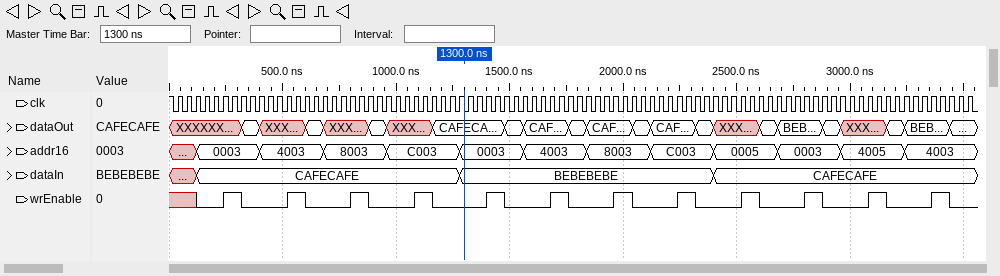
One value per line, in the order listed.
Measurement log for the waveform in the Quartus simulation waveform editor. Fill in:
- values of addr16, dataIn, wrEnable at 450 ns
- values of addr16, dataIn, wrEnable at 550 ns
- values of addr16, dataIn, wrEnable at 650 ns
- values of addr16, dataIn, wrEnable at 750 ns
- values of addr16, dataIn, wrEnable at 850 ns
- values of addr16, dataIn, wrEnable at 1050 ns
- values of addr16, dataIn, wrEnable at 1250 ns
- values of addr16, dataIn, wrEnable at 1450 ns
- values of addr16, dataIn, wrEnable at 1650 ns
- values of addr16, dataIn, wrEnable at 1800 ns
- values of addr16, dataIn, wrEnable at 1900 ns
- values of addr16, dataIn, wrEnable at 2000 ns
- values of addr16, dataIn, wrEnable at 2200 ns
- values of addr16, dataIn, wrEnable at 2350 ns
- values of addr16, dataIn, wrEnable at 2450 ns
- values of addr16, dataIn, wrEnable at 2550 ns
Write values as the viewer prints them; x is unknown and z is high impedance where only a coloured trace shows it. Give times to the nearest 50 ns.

addr16=4003, dataIn=CAFECAFE, wrEnable=0
addr16=4003, dataIn=CAFECAFE, wrEnable=1
addr16=4003, dataIn=CAFECAFE, wrEnable=0
addr16=8003, dataIn=CAFECAFE, wrEnable=0
addr16=8003, dataIn=CAFECAFE, wrEnable=1
addr16=C003, dataIn=CAFECAFE, wrEnable=0
addr16=C003, dataIn=CAFECAFE, wrEnable=0
addr16=0003, dataIn=BEBEBEBE, wrEnable=1
addr16=4003, dataIn=BEBEBEBE, wrEnable=0
addr16=4003, dataIn=BEBEBEBE, wrEnable=0
addr16=8003, dataIn=BEBEBEBE, wrEnable=0
addr16=8003, dataIn=BEBEBEBE, wrEnable=1
addr16=C003, dataIn=BEBEBEBE, wrEnable=0
addr16=C003, dataIn=BEBEBEBE, wrEnable=0
addr16=0005, dataIn=CAFECAFE, wrEnable=0
addr16=0005, dataIn=CAFECAFE, wrEnable=1
